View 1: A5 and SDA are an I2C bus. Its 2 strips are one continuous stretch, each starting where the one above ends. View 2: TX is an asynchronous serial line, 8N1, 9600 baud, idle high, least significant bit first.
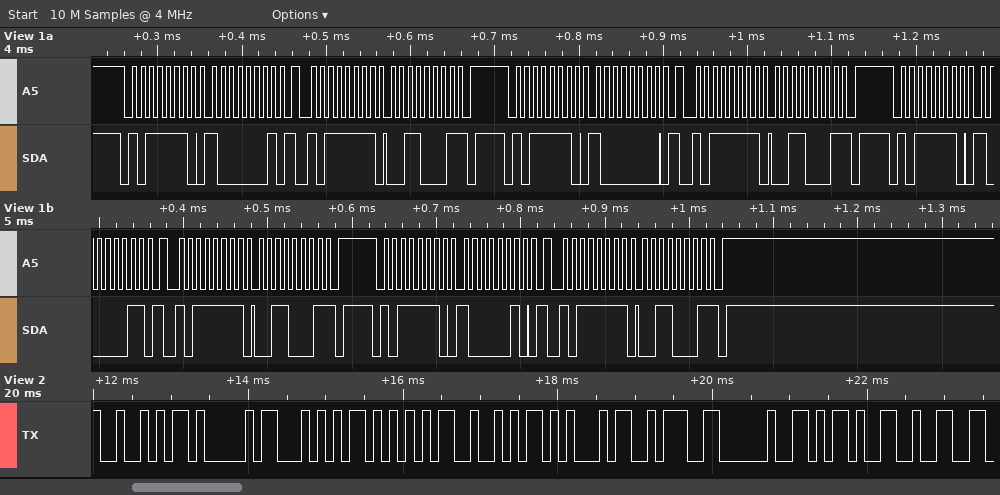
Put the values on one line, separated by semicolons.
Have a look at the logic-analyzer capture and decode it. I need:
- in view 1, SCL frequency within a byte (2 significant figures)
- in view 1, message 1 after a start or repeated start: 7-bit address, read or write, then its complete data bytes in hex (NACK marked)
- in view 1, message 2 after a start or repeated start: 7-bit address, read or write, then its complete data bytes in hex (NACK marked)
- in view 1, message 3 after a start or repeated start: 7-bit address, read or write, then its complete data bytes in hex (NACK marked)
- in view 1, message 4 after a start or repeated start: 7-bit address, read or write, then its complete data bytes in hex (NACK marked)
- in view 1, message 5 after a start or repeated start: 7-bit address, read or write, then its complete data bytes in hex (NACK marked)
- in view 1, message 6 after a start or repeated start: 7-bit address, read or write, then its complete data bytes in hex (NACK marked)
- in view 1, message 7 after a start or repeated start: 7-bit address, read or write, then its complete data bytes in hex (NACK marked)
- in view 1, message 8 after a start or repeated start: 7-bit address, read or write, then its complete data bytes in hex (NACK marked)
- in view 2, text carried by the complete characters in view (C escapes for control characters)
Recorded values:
100 kHz; 0x5F write: 81; 0x5F read: 31 NACK; 0x5F write: 80; 0x5F read: 31 NACK; 0x5F write: 83; 0x5F read: 31 NACK; 0x5F write: 82; 0x5F read: 31 NACK; "RATURE: -2"
